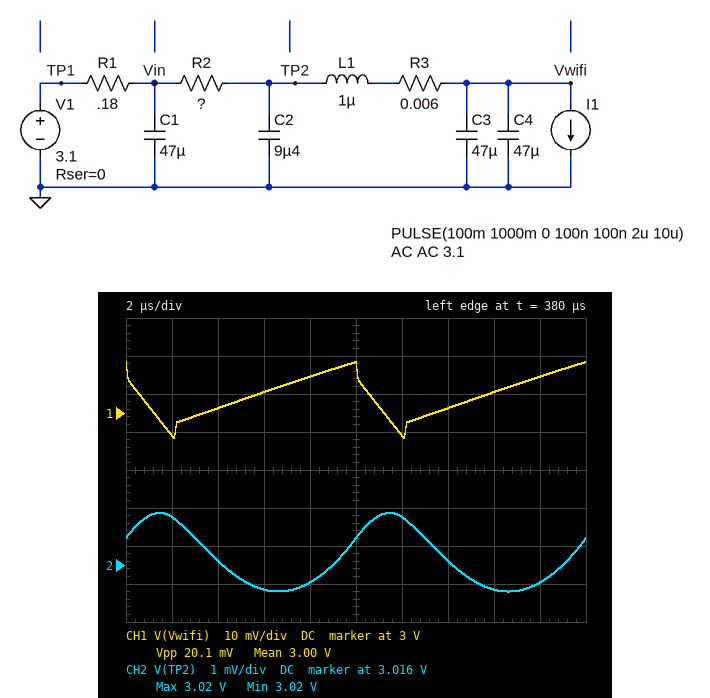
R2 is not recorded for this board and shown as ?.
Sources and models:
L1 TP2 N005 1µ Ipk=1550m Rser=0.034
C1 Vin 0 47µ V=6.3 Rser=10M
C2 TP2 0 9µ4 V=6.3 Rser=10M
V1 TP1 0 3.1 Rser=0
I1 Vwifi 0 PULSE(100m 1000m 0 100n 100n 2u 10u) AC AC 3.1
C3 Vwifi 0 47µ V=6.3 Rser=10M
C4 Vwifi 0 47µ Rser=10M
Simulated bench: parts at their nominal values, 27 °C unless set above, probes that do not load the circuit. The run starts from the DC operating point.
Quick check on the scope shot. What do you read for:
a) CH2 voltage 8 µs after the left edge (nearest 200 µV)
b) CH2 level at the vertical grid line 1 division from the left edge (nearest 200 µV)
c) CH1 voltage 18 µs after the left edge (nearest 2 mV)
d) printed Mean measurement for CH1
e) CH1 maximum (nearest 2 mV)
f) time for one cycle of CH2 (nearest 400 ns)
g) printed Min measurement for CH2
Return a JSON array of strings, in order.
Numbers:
["3.0156 V", "3.0172 V", "3.010 V", "3.00 V", "3.014 V", "10.0 µs", "3.02 V"]
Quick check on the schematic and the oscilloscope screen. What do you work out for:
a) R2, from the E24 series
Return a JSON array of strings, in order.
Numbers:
["0.11 Ω"]
